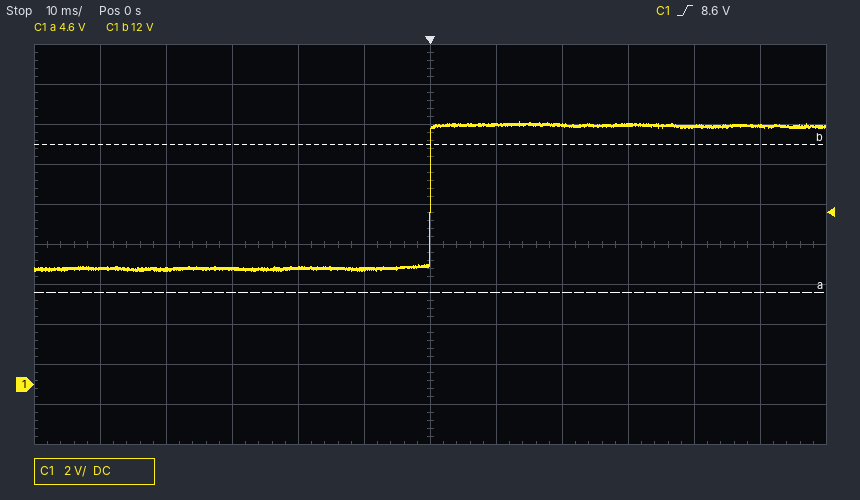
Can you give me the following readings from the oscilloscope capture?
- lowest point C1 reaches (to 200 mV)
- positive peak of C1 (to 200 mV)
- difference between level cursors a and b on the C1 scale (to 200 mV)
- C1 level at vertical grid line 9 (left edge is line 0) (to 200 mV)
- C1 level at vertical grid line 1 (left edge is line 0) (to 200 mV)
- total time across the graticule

5.6 V
13.2 V
7.4 V
13.0 V
5.8 V
120 ms
